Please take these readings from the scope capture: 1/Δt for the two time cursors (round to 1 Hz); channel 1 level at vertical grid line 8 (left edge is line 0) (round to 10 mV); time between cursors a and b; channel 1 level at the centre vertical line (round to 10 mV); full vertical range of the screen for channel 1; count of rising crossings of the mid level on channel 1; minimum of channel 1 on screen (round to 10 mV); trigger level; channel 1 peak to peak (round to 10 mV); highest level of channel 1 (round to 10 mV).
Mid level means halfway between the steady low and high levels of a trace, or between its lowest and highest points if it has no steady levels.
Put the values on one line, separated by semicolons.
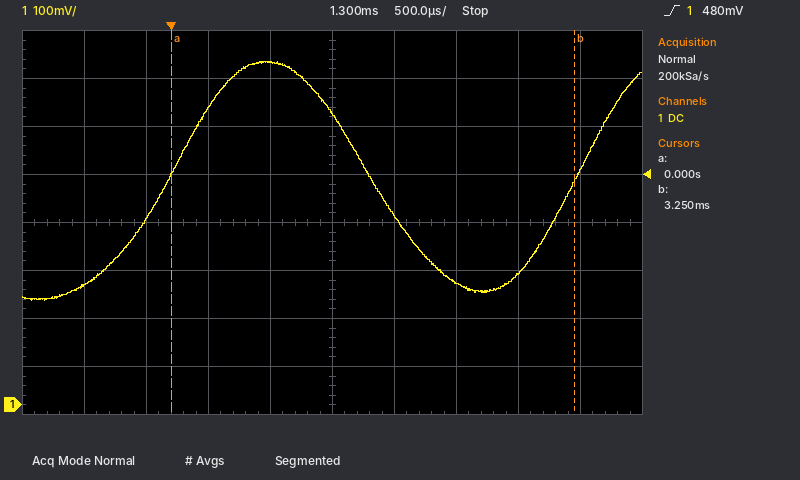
308 Hz; 270 mV; 3.25 ms; 610 mV; 800 mV; 2; 220 mV; 480 mV; 500 mV; 720 mV
